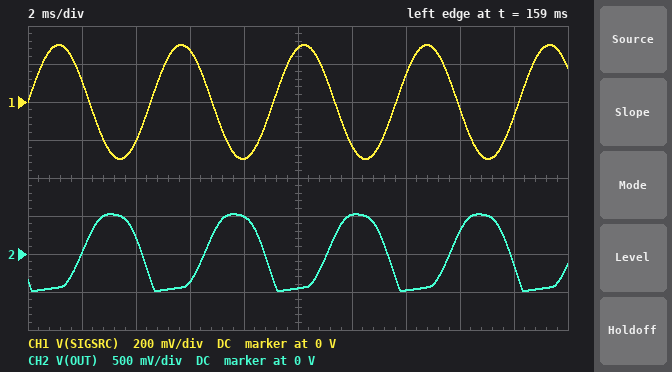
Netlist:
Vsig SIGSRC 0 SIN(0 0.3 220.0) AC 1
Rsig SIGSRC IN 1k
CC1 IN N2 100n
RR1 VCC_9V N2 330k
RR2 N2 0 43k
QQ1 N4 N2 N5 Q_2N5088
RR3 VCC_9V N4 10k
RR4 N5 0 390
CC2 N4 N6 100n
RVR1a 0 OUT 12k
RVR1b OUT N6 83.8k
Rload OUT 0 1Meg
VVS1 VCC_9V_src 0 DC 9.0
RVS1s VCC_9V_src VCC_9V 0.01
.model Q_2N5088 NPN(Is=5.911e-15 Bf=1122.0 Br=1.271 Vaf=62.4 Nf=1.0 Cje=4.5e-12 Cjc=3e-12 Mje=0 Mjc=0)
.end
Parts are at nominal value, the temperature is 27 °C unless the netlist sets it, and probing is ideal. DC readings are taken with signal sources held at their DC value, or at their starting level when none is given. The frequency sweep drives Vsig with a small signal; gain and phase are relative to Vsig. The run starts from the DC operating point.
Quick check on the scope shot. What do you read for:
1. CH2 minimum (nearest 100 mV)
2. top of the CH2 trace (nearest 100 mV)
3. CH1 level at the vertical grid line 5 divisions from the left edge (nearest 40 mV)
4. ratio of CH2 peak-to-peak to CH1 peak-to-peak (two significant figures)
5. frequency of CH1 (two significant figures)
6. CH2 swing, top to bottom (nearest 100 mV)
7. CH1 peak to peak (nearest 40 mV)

-500 mV
500 mV
280 mV
1.7
220 Hz
1.0 V
600 mV
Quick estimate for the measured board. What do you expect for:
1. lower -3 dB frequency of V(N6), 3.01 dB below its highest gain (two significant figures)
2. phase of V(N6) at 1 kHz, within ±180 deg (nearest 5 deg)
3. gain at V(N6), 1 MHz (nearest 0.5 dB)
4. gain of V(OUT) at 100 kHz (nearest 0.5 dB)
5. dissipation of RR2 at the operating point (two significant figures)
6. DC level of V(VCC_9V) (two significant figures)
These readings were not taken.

360 Hz
-160 deg
22.5 dB
5.0 dB
23 µW
9.0 V
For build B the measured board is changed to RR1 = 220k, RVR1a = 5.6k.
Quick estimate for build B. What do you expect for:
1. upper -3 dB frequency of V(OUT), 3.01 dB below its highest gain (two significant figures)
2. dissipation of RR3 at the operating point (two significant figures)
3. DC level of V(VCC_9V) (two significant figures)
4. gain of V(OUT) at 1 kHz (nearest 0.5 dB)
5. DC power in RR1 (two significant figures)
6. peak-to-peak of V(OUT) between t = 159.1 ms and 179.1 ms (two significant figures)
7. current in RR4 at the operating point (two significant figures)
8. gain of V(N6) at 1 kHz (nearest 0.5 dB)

29 MHz
7.3 mW
9.0 V
-27.0 dB
290 µW
350 mV
870 µA
-3.0 dB
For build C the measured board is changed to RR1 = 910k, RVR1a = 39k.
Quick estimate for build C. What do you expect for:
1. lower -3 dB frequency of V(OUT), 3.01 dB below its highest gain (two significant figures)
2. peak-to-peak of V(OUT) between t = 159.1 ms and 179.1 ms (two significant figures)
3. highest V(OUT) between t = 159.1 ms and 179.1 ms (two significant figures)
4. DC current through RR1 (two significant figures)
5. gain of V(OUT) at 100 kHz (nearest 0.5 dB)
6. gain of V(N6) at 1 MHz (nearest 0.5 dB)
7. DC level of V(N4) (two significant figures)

3.9 MHz
530 mV
110 mV
9.4 µA
-43.0 dB
-15.5 dB
9.0 V
